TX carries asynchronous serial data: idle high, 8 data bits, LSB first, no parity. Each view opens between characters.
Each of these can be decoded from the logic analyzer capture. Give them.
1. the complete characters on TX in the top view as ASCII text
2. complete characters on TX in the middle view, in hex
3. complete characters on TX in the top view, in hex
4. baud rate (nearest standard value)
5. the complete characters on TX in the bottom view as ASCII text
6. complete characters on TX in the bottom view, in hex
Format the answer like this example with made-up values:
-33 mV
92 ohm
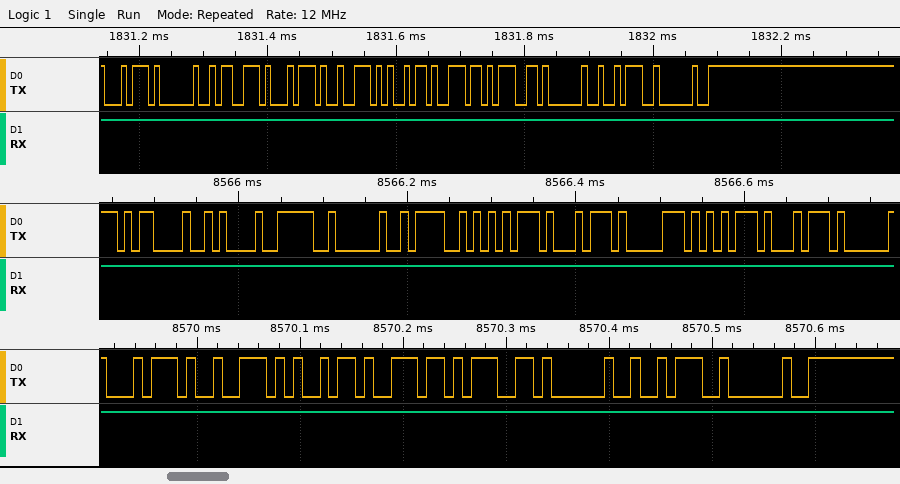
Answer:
"t string : "
0D, 0A, 3E, 20, 4F, 75, 74, 70, 75, 74
74, 20, 73, 74, 72, 69, 6E, 67, 20, 3A, 20
115200 baud
"tring : "
74, 72, 69, 6E, 67, 20, 3A, 20
